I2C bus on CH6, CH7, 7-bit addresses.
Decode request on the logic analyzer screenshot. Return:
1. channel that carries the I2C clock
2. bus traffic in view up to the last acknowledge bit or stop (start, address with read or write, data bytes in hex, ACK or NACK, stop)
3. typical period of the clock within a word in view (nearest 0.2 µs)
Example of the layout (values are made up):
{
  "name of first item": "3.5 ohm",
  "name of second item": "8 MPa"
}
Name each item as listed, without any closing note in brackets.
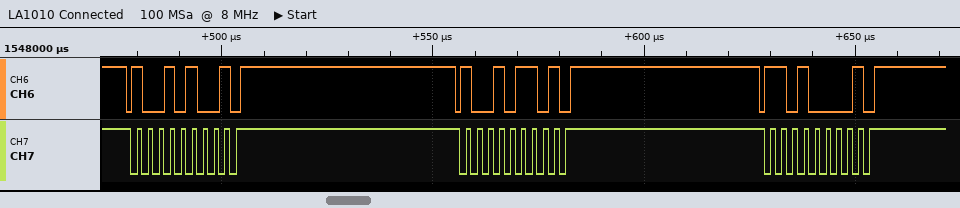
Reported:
{
  "channel that carries the I2C clock": "CH7",
  "bus traffic in view up to the last acknowledge bit or stop": "start, address 4A write NACK, stop, start, address 4B write NACK, stop, start, address 68 write NACK, stop",
  "typical period of the clock within a word in view": "2.6 µs"
}
